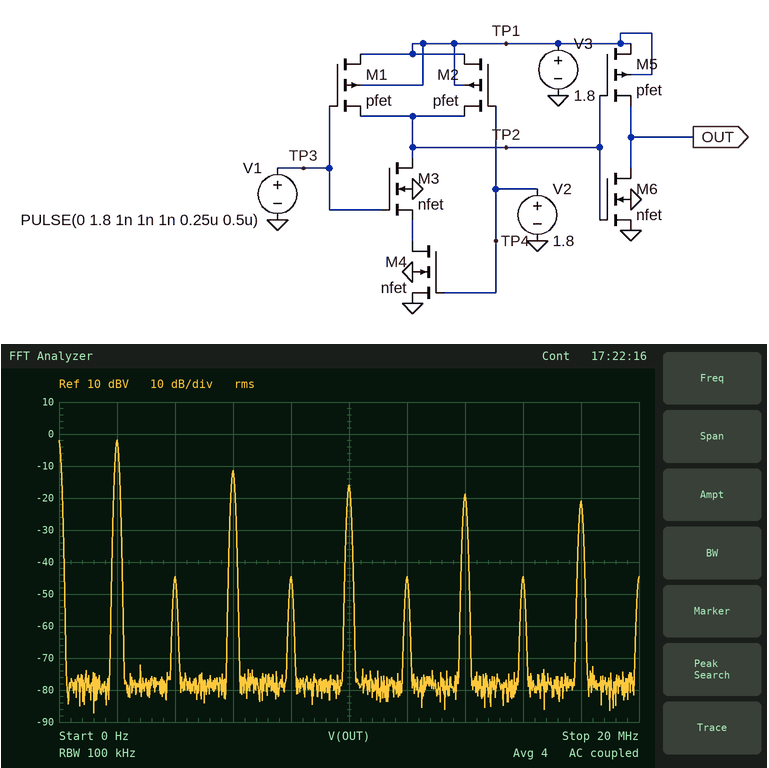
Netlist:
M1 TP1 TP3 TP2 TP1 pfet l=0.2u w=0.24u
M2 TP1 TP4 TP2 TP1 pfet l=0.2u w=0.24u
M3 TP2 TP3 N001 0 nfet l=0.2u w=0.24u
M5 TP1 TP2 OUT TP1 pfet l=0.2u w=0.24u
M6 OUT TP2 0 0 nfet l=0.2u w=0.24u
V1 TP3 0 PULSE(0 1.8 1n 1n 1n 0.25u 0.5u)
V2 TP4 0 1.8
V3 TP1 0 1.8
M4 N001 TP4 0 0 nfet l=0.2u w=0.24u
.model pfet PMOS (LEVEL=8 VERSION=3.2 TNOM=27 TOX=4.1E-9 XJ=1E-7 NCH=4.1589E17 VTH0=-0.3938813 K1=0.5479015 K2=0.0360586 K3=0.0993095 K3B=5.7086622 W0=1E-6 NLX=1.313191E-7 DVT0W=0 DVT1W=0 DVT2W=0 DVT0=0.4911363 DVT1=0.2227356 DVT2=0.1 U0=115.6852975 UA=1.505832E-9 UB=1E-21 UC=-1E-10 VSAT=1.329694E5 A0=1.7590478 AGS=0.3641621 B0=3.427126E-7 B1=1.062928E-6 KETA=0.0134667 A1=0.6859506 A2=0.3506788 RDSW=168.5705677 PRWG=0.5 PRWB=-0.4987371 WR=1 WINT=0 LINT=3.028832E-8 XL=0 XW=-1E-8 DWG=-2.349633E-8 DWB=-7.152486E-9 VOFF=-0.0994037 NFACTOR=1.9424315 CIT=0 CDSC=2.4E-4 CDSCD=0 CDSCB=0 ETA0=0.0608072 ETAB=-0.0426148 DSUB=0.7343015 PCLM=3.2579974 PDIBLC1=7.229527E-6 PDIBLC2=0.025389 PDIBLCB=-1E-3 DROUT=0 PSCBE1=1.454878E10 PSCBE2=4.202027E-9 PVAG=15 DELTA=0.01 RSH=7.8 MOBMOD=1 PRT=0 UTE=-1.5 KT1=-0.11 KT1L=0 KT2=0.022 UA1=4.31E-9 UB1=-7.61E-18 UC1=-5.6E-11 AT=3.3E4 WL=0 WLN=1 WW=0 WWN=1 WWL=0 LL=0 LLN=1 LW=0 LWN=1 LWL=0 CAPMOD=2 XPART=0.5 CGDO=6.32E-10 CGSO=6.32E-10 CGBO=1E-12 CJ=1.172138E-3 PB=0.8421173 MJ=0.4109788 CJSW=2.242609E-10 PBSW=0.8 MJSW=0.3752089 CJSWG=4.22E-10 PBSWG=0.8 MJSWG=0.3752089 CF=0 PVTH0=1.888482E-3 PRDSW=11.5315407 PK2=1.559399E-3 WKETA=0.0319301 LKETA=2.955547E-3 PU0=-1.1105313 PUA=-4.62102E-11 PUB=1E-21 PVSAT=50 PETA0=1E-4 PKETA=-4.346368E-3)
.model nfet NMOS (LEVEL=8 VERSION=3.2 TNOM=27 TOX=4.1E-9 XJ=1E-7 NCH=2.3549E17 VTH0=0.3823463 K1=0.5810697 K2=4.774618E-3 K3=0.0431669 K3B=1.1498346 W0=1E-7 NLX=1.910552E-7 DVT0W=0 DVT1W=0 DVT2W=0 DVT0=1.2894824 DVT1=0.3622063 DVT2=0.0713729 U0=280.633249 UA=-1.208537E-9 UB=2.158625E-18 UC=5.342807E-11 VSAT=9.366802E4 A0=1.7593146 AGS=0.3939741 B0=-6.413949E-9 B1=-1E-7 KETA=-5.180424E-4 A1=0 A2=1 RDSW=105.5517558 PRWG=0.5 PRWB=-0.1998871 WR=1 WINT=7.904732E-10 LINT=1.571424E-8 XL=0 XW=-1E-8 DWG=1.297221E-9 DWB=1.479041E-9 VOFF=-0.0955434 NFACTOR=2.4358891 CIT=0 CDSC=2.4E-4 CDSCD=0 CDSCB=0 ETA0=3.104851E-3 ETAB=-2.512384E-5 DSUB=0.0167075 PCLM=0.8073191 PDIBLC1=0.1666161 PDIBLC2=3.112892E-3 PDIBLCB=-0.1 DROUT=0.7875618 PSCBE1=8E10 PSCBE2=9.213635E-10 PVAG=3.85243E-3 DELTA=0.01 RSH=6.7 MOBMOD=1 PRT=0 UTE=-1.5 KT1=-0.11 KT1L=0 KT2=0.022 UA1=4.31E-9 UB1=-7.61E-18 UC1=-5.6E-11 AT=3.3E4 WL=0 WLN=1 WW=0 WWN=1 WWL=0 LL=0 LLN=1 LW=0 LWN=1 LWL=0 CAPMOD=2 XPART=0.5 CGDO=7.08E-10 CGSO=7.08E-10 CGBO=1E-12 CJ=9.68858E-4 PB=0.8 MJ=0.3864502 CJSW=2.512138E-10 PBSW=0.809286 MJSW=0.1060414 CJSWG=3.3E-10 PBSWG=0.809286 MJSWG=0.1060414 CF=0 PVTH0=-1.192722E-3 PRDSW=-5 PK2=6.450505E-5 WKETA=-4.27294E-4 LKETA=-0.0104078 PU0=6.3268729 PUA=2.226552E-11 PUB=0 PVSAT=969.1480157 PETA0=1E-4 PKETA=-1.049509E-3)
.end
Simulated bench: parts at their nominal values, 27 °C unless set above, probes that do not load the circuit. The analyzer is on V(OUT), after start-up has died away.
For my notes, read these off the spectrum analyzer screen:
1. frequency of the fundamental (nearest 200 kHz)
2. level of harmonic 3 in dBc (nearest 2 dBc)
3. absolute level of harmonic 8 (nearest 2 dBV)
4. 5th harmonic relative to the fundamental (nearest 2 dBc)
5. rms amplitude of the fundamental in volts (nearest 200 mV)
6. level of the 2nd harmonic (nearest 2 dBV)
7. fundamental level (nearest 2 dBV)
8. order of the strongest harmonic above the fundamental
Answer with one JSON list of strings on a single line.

["2.0 MHz", "-10 dBc", "-44 dBV", "-14 dBc", "800 mV", "-44 dBV", "-2 dBV", "3"]
